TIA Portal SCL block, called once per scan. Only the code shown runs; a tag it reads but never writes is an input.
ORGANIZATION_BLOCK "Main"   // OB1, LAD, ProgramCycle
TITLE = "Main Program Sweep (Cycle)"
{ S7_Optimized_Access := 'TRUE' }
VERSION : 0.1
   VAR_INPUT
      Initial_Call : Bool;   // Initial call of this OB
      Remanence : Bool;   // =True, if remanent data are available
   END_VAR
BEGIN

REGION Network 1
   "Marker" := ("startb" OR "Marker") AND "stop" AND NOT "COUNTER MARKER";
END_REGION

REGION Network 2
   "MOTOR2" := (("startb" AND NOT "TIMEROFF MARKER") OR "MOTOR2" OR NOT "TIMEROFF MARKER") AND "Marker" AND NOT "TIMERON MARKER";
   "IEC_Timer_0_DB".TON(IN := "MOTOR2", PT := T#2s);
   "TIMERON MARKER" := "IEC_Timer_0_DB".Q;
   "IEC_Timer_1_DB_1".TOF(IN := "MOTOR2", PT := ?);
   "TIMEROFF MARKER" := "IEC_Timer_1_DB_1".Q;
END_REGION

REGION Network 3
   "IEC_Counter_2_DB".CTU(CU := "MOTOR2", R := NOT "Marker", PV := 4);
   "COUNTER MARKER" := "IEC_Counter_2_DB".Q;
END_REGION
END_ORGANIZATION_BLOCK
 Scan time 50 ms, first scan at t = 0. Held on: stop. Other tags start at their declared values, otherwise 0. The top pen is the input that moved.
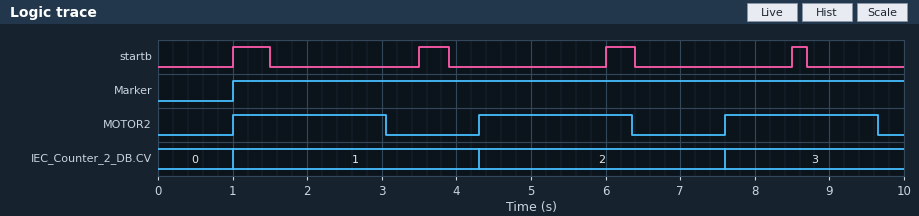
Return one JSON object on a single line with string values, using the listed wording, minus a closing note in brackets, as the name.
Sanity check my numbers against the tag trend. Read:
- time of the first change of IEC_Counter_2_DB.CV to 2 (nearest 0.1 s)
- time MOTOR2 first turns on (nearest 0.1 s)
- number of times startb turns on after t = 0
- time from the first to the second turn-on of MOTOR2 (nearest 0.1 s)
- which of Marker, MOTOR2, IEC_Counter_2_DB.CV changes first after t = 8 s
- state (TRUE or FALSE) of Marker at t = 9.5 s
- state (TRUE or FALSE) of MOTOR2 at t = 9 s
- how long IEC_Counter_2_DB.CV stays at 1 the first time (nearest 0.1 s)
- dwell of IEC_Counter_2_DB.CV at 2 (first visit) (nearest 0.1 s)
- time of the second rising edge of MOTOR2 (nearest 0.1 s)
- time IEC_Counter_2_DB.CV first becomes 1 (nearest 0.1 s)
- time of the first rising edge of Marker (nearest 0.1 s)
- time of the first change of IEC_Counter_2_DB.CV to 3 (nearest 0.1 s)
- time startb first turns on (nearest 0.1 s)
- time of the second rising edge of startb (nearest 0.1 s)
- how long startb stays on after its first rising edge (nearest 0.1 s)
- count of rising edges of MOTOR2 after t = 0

{"time of the first change of IEC_Counter_2_DB.CV to 2": "4.3 s", "time MOTOR2 first turns on": "1.0 s", "number of times startb turns on after t = 0": "4", "time from the first to the second turn-on of MOTOR2": "3.3 s", "which of Marker, MOTOR2, IEC_Counter_2_DB.CV changes first after t = 8 s": "MOTOR2", "state (TRUE or FALSE) of Marker at t = 9.5 s": "TRUE", "state (TRUE or FALSE) of MOTOR2 at t = 9 s": "TRUE", "how long IEC_Counter_2_DB.CV stays at 1 the first time": "3.3 s", "dwell of IEC_Counter_2_DB.CV at 2 (first visit)": "3.3 s", "time of the second rising edge of MOTOR2": "4.3 s", "time IEC_Counter_2_DB.CV first becomes 1": "1.0 s", "time of the first rising edge of Marker": "1.0 s", "time of the first change of IEC_Counter_2_DB.CV to 3": "7.6 s", "time startb first turns on": "1.0 s", "time of the second rising edge of startb": "3.5 s", "how long startb stays on after its first rising edge": "0.5 s", "count of rising edges of MOTOR2 after t = 0": "3"}
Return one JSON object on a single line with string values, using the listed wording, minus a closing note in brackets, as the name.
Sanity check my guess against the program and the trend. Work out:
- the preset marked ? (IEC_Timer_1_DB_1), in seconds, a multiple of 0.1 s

{"the preset marked ? (IEC_Timer_1_DB_1), in seconds, a multiple of 0.1 s": "1.2 s"}
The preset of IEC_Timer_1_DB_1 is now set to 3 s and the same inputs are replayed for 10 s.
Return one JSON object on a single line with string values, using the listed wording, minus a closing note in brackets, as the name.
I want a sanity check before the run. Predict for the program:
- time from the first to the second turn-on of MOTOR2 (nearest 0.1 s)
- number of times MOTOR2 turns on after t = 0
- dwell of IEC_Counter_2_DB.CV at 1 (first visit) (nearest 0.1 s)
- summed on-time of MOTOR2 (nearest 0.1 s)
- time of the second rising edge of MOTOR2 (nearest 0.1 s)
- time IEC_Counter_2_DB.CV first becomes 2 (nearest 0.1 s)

{"time from the first to the second turn-on of MOTOR2": "5.1 s", "number of times MOTOR2 turns on after t = 0": "2", "dwell of IEC_Counter_2_DB.CV at 1 (first visit)": "5.1 s", "summed on-time of MOTOR2": "4.1 s", "time of the second rising edge of MOTOR2": "6.1 s", "time IEC_Counter_2_DB.CV first becomes 2": "6.1 s"}
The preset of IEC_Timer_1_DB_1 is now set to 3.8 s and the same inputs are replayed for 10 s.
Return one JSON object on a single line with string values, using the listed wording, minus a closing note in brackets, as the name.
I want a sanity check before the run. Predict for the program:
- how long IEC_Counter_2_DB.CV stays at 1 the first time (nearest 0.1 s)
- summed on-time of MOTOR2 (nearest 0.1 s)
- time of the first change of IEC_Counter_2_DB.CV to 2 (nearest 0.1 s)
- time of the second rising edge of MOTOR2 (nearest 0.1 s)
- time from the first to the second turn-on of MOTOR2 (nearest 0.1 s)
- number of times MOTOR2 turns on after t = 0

{"how long IEC_Counter_2_DB.CV stays at 1 the first time": "5.9 s", "summed on-time of MOTOR2": "4.1 s", "time of the first change of IEC_Counter_2_DB.CV to 2": "6.9 s", "time of the second rising edge of MOTOR2": "6.9 s", "time from the first to the second turn-on of MOTOR2": "5.9 s", "number of times MOTOR2 turns on after t = 0": "2"}
